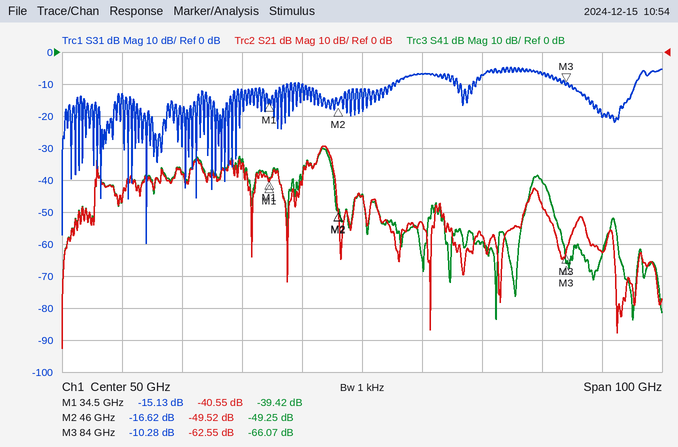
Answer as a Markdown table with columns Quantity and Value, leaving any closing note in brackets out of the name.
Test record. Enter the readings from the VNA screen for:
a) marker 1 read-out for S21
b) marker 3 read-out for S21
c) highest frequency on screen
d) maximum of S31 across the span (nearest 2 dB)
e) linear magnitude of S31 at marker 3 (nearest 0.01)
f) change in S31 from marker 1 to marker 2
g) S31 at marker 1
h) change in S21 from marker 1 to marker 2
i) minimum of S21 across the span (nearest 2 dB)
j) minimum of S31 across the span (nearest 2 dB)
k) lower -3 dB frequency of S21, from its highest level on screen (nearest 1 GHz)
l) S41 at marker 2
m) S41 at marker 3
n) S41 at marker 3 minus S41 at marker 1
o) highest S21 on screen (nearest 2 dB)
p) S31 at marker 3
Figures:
| Quantity | Value |
|---|---|
| marker 1 read-out for S21 | -40.55 dB |
| marker 3 read-out for S21 | -62.55 dB |
| highest frequency on screen | 100 GHz |
| maximum of S31 across the span | -4 dB |
| linear magnitude of S31 at marker 3 | 0.31 |
| change in S31 from marker 1 to marker 2 | -1.49 dB |
| S31 at marker 1 | -15.13 dB |
| change in S21 from marker 1 to marker 2 | -8.97 dB |
| minimum of S21 across the span | -92 dB |
| minimum of S31 across the span | -60 dB |
| lower -3 dB frequency of S21, from its highest level on screen | 43 GHz |
| S41 at marker 2 | -49.25 dB |
| S41 at marker 3 | -66.07 dB |
| S41 at marker 3 minus S41 at marker 1 | -26.65 dB |
| highest S21 on screen | -30 dB |
| S31 at marker 3 | -10.28 dB |
